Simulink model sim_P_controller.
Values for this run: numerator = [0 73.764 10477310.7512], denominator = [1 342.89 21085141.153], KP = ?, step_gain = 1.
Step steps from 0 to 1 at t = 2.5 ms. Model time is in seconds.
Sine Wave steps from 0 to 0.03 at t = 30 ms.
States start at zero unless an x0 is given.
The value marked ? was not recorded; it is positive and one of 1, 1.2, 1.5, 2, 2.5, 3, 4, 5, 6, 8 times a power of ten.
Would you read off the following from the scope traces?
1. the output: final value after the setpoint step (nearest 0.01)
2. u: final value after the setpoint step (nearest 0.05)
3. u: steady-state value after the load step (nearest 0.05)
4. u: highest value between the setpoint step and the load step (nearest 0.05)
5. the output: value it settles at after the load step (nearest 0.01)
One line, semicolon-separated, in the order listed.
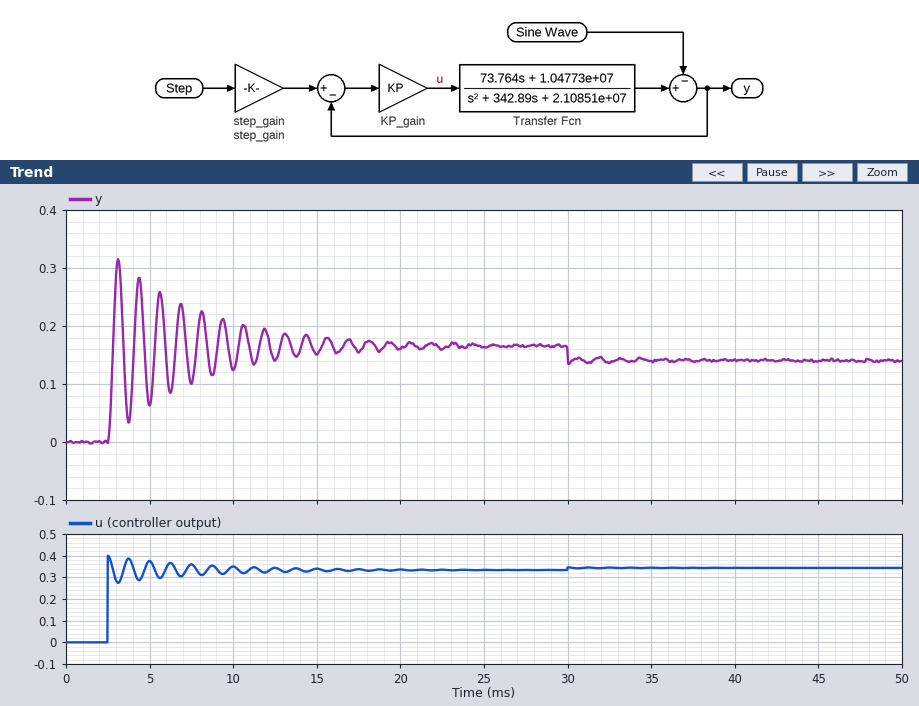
0.17; 0.35; 0.35; 0.40; 0.14
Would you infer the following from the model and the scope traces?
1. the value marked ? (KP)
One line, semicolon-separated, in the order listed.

0.4
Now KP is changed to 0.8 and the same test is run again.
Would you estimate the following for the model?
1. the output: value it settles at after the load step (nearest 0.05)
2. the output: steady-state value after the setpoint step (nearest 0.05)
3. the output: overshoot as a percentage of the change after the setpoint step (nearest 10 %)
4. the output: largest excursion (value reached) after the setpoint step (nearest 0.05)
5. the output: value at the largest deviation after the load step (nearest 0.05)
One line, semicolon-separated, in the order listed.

0.25; 0.30; 90 %; 0.55; 0.25
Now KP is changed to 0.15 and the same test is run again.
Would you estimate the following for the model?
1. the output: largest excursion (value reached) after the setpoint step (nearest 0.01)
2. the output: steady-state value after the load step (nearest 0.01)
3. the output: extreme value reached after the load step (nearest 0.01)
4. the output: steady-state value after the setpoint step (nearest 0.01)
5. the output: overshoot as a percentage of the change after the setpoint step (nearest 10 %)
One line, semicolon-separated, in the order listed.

0.13; 0.04; 0.04; 0.07; 90 %
